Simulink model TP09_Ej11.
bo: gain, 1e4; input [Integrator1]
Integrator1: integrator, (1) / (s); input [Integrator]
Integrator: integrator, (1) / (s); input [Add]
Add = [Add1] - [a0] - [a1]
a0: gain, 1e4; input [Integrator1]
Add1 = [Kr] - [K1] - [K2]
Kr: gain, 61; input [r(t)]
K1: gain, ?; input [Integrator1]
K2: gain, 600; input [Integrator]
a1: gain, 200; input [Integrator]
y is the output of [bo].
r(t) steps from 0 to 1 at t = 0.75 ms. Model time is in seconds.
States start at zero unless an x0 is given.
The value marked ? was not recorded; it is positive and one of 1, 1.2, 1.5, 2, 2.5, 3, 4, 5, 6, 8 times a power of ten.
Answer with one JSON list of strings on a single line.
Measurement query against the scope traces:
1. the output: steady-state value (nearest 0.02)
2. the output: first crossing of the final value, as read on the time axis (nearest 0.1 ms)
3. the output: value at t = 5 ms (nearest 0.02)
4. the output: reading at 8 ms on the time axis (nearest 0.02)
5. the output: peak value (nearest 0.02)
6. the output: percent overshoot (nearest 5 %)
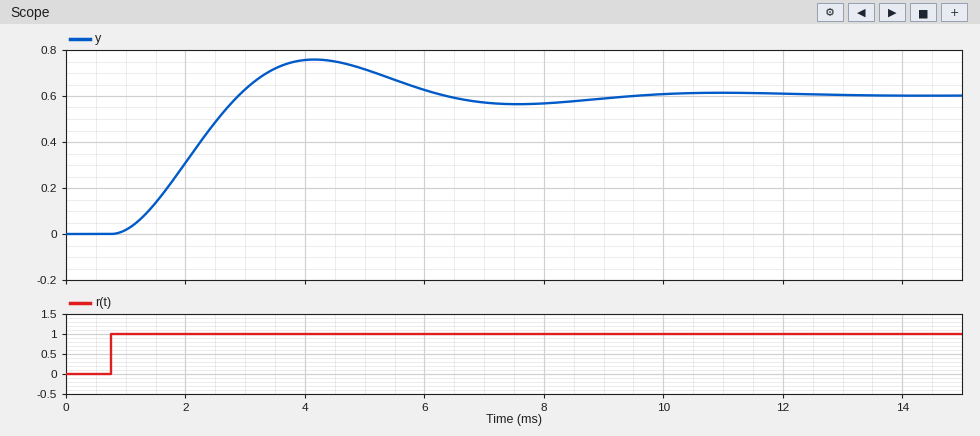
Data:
["0.60", "2.9 ms", "0.72", "0.56", "0.76", "25 %"]
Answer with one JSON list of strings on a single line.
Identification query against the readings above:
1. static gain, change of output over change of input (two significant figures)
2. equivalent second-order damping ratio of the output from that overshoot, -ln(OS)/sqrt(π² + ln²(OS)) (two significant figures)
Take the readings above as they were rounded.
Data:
["0.60", "0.40"]
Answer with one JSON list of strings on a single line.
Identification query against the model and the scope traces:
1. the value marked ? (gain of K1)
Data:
["1e+06"]
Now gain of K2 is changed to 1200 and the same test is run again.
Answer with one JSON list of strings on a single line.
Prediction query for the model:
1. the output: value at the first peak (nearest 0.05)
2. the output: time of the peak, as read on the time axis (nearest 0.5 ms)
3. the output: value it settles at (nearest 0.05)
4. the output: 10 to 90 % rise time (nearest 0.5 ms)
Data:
["0.65", "5.0 ms", "0.60", "2.0 ms"]
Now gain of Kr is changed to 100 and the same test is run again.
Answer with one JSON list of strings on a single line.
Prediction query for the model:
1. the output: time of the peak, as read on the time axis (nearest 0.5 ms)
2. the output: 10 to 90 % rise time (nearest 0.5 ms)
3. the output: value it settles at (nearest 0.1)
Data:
["4.0 ms", "1.5 ms", "1.0"]
